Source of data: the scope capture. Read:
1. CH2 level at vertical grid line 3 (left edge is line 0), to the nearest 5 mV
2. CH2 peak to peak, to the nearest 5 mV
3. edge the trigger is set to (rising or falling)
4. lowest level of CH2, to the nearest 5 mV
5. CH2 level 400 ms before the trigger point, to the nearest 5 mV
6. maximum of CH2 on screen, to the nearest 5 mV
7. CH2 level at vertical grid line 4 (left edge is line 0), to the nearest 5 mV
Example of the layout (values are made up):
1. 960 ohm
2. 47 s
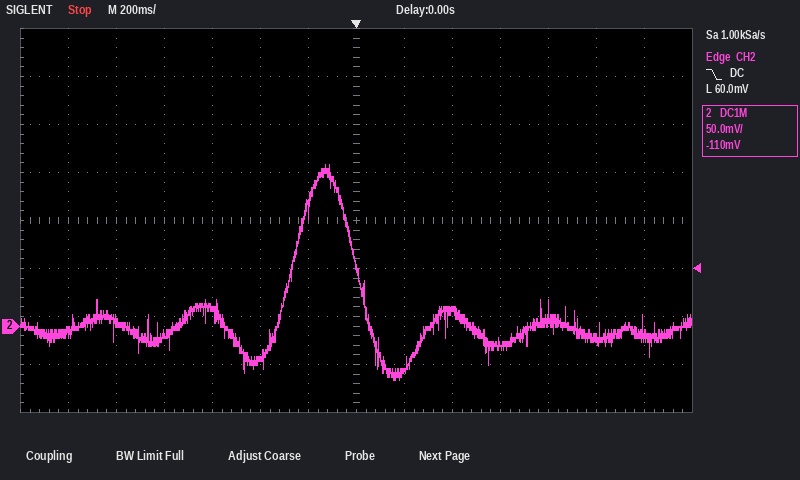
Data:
1. -10 mV
2. 225 mV
3. falling
4. -55 mV
5. -35 mV
6. 170 mV
7. 20 mV
